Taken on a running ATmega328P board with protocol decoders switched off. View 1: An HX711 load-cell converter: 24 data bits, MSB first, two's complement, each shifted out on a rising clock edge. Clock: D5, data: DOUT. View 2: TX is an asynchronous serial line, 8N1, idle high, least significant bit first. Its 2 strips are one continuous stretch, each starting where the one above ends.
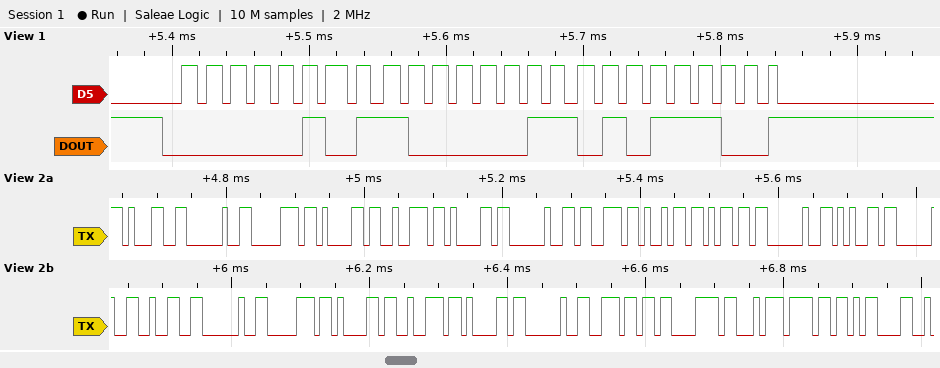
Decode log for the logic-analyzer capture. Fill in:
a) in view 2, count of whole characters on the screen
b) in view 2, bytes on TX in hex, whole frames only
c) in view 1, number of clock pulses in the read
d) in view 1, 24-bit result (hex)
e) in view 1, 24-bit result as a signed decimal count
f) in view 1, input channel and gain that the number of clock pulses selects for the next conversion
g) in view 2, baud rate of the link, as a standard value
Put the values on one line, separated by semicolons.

25; 0x31 0x20 0x70 0x61 0x72 0x61 0x20 0x73 0x69 0x6D 0x20 0x65 0x20 0x32 0x20 0x70 0x61 0x72 0x61 0x20 0x6E 0xC3 0xA3 0x6F 0x0D; 25; 0x05835C; 361308; channel A, gain 128; 115200 baud
